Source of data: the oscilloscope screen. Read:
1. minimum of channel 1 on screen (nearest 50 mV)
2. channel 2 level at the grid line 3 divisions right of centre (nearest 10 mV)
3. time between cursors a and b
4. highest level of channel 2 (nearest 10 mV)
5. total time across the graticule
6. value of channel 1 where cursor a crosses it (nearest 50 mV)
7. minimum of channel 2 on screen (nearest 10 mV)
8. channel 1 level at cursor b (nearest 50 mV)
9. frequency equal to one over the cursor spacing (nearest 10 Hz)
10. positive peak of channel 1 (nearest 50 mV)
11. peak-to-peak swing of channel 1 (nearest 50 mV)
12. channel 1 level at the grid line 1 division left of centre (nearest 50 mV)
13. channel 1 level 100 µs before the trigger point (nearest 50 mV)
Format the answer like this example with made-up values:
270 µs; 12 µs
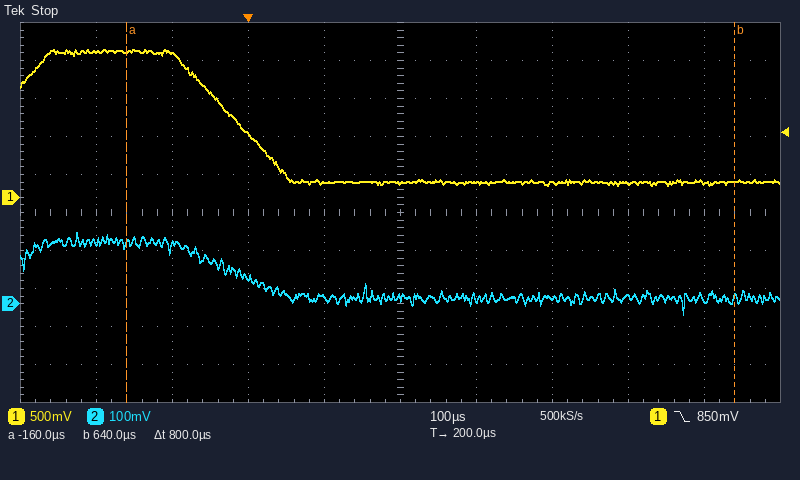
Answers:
150 mV; 20 mV; 800 µs; 190 mV; 1 ms; 1.90 V; -30 mV; 200 mV; 1.25 kHz; 1.95 V; 1.80 V; 200 mV; 1.90 V
